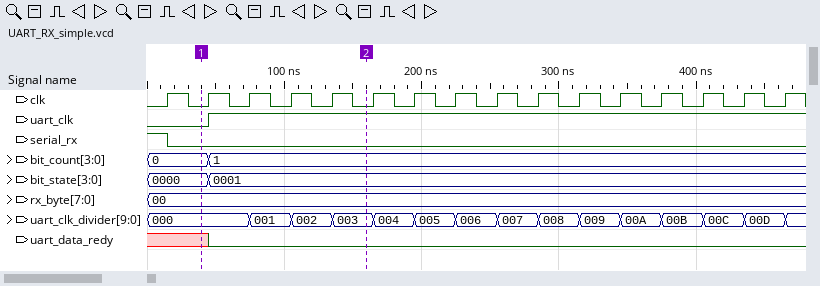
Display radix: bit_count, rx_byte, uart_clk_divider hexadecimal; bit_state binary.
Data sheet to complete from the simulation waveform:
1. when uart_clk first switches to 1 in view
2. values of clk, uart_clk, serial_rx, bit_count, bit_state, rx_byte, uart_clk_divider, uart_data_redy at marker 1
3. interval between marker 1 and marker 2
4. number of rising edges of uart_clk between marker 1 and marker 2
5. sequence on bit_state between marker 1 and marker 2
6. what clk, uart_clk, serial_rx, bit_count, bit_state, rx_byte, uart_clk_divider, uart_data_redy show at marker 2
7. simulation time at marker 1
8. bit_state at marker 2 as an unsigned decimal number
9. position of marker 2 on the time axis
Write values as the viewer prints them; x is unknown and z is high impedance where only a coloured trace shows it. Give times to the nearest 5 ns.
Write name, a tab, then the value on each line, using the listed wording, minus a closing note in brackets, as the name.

when uart_clk first switches to 1 in view	45 ns
values of clk, uart_clk, serial_rx, bit_count, bit_state, rx_byte, uart_clk_divider, uart_data_redy at marker 1	clk=0, uart_clk=0, serial_rx=0, bit_count=0, bit_state=0000, rx_byte=00, uart_clk_divider=000, uart_data_redy=x
interval between marker 1 and marker 2	120 ns
number of rising edges of uart_clk between marker 1 and marker 2	1
sequence on bit_state between marker 1 and marker 2	0000, 0001
what clk, uart_clk, serial_rx, bit_count, bit_state, rx_byte, uart_clk_divider, uart_data_redy show at marker 2	clk=0, uart_clk=1, serial_rx=0, bit_count=1, bit_state=0001, rx_byte=00, uart_clk_divider=003, uart_data_redy=0
simulation time at marker 1	40 ns
bit_state at marker 2 as an unsigned decimal number	1
position of marker 2 on the time axis	160 ns
